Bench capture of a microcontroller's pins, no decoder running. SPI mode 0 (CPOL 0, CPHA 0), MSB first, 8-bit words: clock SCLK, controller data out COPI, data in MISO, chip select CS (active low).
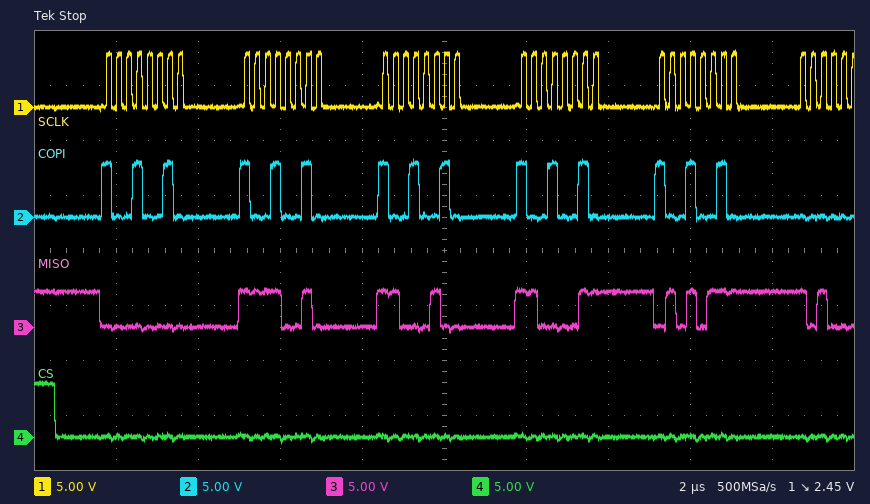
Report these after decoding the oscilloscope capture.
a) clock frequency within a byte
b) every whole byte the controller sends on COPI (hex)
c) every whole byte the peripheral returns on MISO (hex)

4 MHz
92 92 92 92 92
00 F2 C4 C3 57
